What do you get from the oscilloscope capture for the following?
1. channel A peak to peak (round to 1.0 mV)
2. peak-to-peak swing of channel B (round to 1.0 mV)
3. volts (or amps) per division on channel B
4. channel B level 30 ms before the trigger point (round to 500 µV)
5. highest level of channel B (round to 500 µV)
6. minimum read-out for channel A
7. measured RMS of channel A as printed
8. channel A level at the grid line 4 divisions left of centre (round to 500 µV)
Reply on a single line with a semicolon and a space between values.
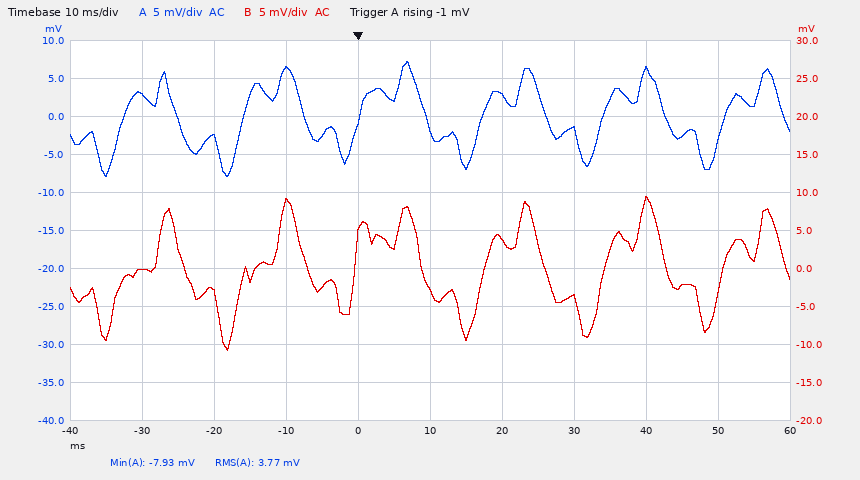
15.0 mV; 20.0 mV; 5 mV; 0.0 mV; 9.5 mV; -7.93 mV; 3.77 mV; 3.0 mV
